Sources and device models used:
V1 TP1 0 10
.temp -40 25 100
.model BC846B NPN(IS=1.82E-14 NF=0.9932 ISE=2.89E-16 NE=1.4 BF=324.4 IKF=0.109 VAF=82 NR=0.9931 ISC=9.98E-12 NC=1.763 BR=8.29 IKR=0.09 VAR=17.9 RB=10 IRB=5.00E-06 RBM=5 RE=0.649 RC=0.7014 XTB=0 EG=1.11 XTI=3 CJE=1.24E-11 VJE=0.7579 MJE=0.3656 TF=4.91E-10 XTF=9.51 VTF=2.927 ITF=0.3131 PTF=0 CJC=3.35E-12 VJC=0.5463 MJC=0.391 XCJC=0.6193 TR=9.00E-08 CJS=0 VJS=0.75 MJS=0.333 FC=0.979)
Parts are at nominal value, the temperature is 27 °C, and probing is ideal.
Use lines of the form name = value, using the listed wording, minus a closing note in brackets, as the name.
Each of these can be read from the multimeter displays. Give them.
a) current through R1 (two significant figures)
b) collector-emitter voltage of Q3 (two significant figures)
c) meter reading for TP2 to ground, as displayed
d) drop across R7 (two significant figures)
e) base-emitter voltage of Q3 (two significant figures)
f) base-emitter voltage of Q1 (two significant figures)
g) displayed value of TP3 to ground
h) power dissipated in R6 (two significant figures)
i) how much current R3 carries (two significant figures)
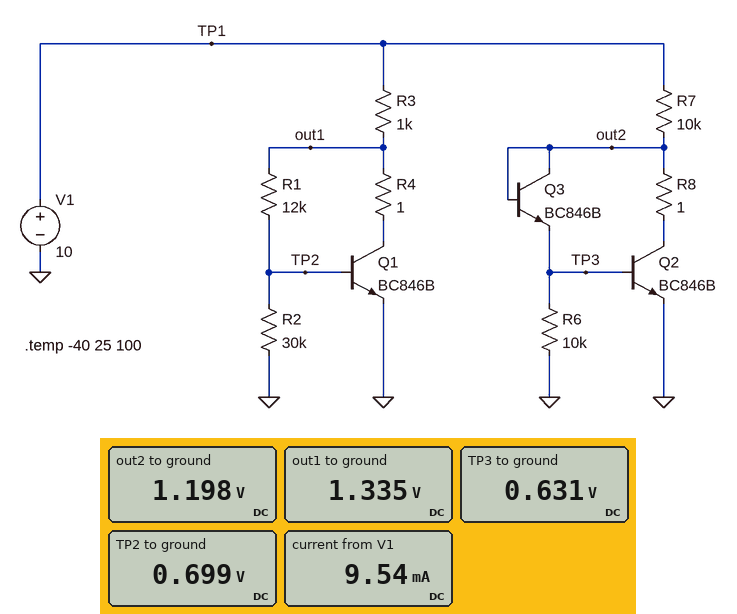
current through R1 = 53 µA
collector-emitter voltage of Q3 = 570 mV
meter reading for TP2 to ground, as displayed = 0.699 V
drop across R7 = 8.8 V
base-emitter voltage of Q3 = 570 mV
base-emitter voltage of Q1 = 700 mV
displayed value of TP3 to ground = 0.631 V
power dissipated in R6 = 40 µW
how much current R3 carries = 8.7 mA
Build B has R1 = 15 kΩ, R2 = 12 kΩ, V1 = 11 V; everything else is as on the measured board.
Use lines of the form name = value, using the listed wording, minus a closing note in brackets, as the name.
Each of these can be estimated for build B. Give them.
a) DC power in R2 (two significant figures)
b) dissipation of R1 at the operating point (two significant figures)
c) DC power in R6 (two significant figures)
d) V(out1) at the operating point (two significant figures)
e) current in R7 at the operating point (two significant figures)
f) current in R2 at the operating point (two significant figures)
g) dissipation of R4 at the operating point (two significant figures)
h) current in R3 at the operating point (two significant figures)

DC power in R2 = 41 µW
dissipation of R1 at the operating point = 120 µW
DC power in R6 = 40 µW
V(out1) at the operating point = 2.0 V
current in R7 at the operating point = 980 µA
current in R2 at the operating point = 58 µA
dissipation of R4 at the operating point = 79 µW
current in R3 at the operating point = 9.0 mA
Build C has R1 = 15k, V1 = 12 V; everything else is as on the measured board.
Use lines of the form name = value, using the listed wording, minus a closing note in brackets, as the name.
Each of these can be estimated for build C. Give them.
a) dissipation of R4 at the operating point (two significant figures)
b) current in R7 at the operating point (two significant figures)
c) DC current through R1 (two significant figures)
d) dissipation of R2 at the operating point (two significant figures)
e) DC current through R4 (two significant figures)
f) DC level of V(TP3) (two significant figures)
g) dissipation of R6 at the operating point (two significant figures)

dissipation of R4 at the operating point = 110 µW
current in R7 at the operating point = 1.1 mA
DC current through R1 = 60 µA
dissipation of R2 at the operating point = 17 µW
DC current through R4 = 10 mA
DC level of V(TP3) = 640 mV
dissipation of R6 at the operating point = 41 µW
